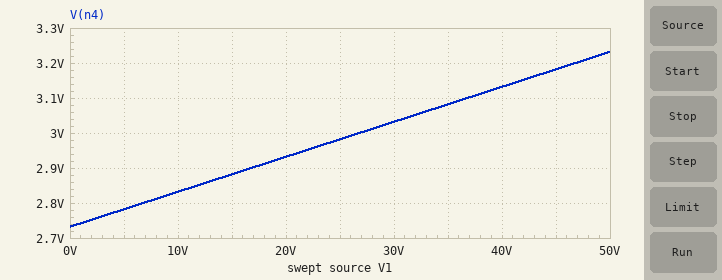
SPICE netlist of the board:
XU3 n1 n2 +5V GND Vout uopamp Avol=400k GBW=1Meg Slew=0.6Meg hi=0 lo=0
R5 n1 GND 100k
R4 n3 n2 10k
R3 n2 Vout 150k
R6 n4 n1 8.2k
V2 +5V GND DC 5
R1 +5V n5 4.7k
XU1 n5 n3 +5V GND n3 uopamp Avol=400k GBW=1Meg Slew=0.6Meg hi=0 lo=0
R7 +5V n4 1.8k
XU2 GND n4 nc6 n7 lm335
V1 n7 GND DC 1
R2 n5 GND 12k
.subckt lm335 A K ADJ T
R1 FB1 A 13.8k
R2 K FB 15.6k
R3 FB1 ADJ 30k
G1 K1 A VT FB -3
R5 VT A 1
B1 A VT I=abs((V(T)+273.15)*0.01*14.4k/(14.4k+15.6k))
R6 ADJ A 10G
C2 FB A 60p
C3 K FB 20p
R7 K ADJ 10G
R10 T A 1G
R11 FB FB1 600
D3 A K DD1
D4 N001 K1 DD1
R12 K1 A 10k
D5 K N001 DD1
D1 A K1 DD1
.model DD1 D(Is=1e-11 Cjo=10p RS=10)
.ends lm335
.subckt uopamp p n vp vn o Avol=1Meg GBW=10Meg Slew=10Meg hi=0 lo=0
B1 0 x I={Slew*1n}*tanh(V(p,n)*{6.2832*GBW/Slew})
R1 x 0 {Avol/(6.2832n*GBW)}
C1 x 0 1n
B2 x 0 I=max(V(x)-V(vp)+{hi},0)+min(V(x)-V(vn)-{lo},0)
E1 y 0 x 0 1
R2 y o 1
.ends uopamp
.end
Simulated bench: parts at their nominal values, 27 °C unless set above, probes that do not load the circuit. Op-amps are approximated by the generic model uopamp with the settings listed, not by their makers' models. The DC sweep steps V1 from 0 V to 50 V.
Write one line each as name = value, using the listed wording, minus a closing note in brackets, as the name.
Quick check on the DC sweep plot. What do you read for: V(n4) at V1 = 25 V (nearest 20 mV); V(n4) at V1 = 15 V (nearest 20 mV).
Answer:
V(n4) at V1 = 25 V = 2.98 V
V(n4) at V1 = 15 V = 2.88 V
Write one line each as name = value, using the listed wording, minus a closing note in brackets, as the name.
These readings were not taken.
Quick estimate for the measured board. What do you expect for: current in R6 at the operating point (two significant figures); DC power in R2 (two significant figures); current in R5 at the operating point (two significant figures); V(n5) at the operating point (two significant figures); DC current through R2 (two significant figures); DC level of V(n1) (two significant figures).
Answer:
current in R6 at the operating point = 25 µA
DC power in R2 = 1.1 mW
current in R5 at the operating point = 25 µA
V(n5) at the operating point = 3.6 V
DC current through R2 = 300 µA
DC level of V(n1) = 2.5 V
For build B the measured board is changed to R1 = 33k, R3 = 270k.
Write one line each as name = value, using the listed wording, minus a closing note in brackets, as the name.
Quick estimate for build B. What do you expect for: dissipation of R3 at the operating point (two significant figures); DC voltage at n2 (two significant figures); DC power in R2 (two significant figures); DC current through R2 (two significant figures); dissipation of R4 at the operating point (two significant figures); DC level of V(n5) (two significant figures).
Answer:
dissipation of R3 at the operating point = 46 µW
DC voltage at n2 = 1.5 V
DC power in R2 = 150 µW
DC current through R2 = 110 µA
dissipation of R4 at the operating point = 1.7 µW
DC level of V(n5) = 1.3 V
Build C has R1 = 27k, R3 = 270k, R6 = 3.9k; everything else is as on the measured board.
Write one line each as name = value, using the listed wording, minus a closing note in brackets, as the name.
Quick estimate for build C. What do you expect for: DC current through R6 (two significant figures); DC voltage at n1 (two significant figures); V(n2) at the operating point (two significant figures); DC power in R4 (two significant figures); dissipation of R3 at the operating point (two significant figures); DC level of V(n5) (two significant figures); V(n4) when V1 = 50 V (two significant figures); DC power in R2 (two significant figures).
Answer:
DC current through R6 = 26 µA
DC voltage at n1 = 2.6 V
V(n2) at the operating point = 1.7 V
DC power in R4 = 1.5 µW
dissipation of R3 at the operating point = 41 µW
DC level of V(n5) = 1.5 V
V(n4) when V1 = 50 V = 3.2 V
DC power in R2 = 200 µW
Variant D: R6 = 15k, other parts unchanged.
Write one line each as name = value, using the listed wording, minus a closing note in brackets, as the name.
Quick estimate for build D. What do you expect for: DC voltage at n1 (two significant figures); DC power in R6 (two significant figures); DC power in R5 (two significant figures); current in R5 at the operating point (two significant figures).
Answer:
DC voltage at n1 = 2.4 V
DC power in R6 = 8.5 µW
DC power in R5 = 57 µW
current in R5 at the operating point = 24 µA
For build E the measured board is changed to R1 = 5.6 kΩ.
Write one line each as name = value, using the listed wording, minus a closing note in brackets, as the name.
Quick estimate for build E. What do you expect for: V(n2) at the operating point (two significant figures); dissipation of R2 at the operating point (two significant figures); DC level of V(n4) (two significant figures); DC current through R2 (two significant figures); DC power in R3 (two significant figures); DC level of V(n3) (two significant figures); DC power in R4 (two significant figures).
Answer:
V(n2) at the operating point = 3.2 V
dissipation of R2 at the operating point = 970 µW
DC level of V(n4) = 2.7 V
DC current through R2 = 280 µA
DC power in R3 = 68 µW
DC level of V(n3) = 3.4 V
DC power in R4 = 4.5 µW
